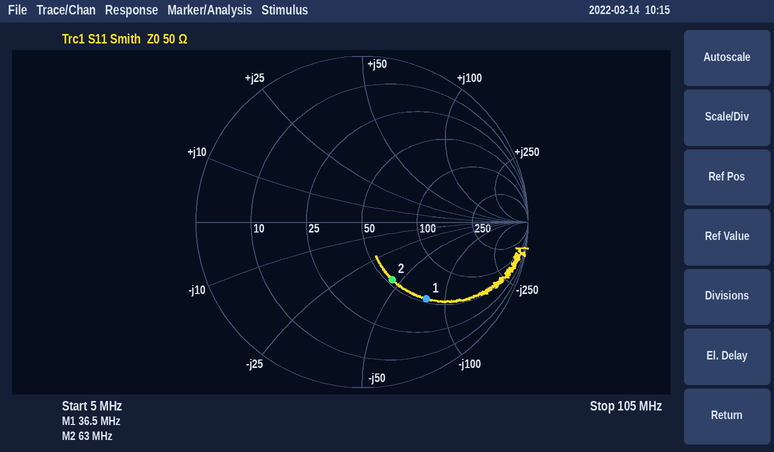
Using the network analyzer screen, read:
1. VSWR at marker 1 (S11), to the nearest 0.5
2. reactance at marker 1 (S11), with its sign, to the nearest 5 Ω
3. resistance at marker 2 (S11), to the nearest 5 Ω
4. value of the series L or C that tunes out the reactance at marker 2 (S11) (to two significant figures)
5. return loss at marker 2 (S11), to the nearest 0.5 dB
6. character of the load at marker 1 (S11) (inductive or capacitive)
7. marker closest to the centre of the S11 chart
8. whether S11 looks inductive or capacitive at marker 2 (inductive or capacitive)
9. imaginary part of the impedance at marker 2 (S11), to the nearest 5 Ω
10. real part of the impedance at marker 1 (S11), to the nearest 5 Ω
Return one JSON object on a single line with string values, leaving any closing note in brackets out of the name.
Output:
{"VSWR at marker 1 (S11), to the nearest 0.5": "4.0", "reactance at marker 1 (S11), with its sign, to the nearest 5 Ω": "-80 Ω", "resistance at marker 2 (S11), to the nearest 5 Ω": "55 Ω", "value of the series L or C that tunes out the reactance at marker 2 (S11)": "110 nH", "return loss at marker 2 (S11), to the nearest 0.5 dB": "8.0 dB", "character of the load at marker 1 (S11)": "capacitive", "marker closest to the centre of the S11 chart": "marker 2", "whether S11 looks inductive or capacitive at marker 2": "capacitive", "imaginary part of the impedance at marker 2 (S11), to the nearest 5 Ω": "-45 Ω", "real part of the impedance at marker 1 (S11), to the nearest 5 Ω": "55 Ω"}
